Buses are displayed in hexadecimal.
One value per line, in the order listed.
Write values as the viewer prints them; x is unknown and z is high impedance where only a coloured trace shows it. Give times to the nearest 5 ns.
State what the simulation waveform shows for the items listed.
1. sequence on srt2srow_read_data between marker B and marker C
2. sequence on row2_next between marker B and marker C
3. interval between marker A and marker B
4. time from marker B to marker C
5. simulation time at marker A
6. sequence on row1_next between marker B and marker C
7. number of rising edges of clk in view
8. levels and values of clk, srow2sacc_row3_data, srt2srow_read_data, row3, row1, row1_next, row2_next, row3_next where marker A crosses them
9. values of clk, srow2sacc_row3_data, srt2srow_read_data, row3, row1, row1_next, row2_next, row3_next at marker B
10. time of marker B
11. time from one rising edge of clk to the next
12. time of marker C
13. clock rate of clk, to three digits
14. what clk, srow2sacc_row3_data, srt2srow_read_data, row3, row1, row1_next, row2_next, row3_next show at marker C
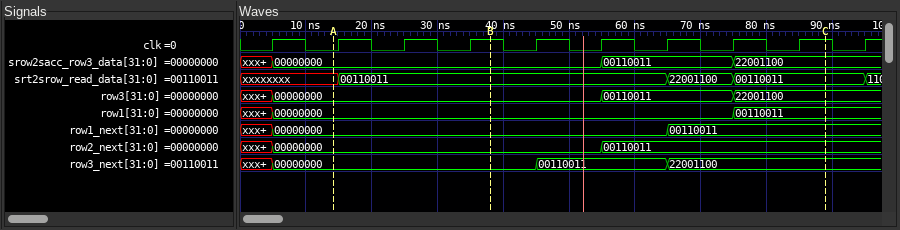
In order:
00110011, 22001100, 00110011
00000000, 00110011
25 ns
50 ns
15 ns
00000000, 00110011
10
clk=0, srow2sacc_row3_data=00000000, srt2srow_read_data=xxxxxxxx, row3=00000000, row1=00000000, row1_next=00000000, row2_next=00000000, row3_next=00000000
clk=1, srow2sacc_row3_data=00000000, srt2srow_read_data=00110011, row3=00000000, row1=00000000, row1_next=00000000, row2_next=00000000, row3_next=00000000
40 ns
10 ns
90 ns
100 MHz
clk=1, srow2sacc_row3_data=22001100, srt2srow_read_data=00110011, row3=22001100, row1=00110011, row1_next=00110011, row2_next=00110011, row3_next=22001100
